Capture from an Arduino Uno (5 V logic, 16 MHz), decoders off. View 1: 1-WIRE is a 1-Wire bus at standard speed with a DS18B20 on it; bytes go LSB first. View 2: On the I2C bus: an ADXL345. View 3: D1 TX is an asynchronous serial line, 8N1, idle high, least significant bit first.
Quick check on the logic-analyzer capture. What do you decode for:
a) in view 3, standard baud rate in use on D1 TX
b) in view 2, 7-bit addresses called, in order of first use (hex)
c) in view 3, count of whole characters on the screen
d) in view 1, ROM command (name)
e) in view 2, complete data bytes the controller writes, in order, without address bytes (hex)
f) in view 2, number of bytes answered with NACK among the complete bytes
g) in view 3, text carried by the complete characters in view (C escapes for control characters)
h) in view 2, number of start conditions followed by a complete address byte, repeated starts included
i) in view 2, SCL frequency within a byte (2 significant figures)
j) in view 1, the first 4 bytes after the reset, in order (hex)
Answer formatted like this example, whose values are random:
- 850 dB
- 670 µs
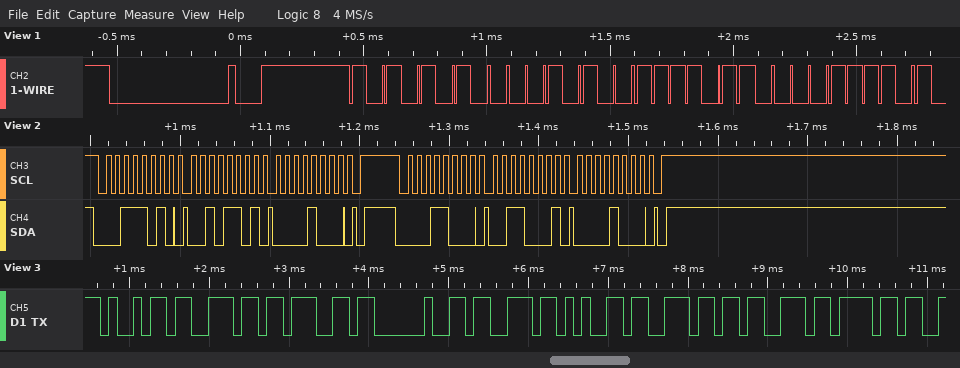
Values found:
- 9600 baud
- 0x1D 0x0C
- 9
- Match ROM
- 2D 08 31 08
- 0
- "ing senso"
- 2
- 100 kHz
- 55 28 6F 78
